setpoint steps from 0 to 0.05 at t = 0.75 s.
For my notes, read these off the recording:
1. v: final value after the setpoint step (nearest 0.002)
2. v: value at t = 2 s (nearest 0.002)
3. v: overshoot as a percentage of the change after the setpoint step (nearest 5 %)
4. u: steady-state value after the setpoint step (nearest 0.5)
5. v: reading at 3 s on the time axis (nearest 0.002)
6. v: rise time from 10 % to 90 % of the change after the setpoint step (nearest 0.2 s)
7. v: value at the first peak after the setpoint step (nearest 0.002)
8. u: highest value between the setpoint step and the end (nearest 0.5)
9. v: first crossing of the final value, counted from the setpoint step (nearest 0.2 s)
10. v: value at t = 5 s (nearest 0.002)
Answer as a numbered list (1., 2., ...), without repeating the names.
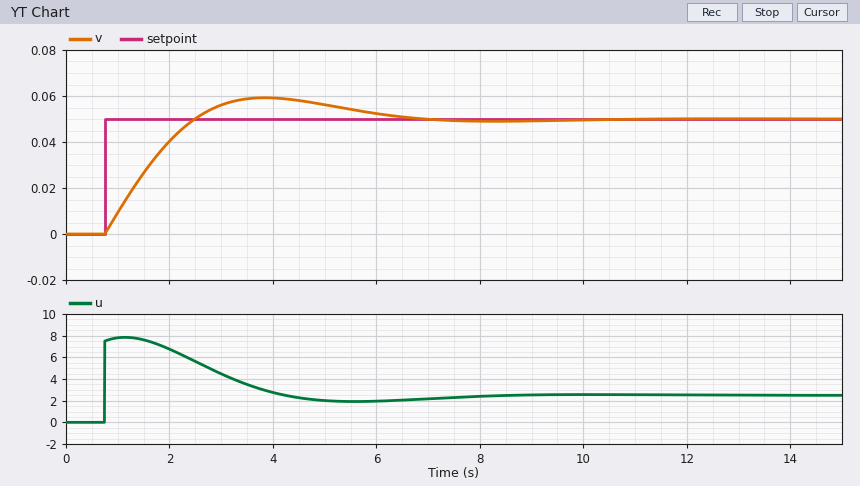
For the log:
1. 0.050
2. 0.040
3. 20 %
4. 2.5
5. 0.056
6. 1.4 s
7. 0.060
8. 8.0
9. 1.8 s
10. 0.056
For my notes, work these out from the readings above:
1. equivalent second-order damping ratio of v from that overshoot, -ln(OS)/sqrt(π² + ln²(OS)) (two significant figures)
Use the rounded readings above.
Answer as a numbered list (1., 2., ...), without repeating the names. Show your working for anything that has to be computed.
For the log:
1. ln(0.2) = -1.609; 1.609 / sqrt(9.870 + 2.590) = 0.46
